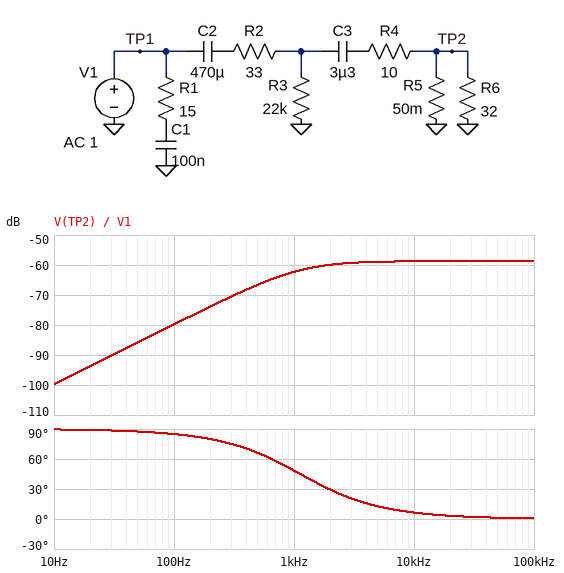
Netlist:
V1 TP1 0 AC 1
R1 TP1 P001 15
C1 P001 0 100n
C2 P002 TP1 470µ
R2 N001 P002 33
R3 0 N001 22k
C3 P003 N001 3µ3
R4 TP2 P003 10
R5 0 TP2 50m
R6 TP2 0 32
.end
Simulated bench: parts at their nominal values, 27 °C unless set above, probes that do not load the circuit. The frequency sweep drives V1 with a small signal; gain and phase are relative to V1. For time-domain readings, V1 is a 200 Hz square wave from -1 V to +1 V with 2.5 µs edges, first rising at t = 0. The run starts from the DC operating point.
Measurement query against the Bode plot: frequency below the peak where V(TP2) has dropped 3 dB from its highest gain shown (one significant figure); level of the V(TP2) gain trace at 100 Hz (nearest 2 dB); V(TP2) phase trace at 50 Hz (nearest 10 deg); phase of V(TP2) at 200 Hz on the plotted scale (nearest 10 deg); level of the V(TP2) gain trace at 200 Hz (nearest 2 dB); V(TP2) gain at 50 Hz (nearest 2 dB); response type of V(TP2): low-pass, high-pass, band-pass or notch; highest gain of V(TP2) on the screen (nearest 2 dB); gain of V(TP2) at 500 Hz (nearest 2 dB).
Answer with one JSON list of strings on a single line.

["1 kHz", "-80 dB", "90 deg", "80 deg", "-74 dB", "-86 dB", "high-pass", "-58 dB", "-66 dB"]
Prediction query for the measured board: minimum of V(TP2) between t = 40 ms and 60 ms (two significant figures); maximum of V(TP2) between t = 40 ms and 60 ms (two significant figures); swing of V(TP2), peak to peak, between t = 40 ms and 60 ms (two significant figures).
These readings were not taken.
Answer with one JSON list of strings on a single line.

["-2.3 mV", "2.3 mV", "4.6 mV"]
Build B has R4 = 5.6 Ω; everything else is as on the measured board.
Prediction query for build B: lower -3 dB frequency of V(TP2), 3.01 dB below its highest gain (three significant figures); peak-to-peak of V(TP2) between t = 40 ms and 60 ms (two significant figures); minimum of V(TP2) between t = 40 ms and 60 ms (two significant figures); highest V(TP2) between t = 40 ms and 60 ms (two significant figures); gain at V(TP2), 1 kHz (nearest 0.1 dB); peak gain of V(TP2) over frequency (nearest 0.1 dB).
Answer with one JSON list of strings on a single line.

["1.26 kHz", "5.1 mV", "-2.6 mV", "2.6 mV", "-61.9 dB", "-57.8 dB"]
